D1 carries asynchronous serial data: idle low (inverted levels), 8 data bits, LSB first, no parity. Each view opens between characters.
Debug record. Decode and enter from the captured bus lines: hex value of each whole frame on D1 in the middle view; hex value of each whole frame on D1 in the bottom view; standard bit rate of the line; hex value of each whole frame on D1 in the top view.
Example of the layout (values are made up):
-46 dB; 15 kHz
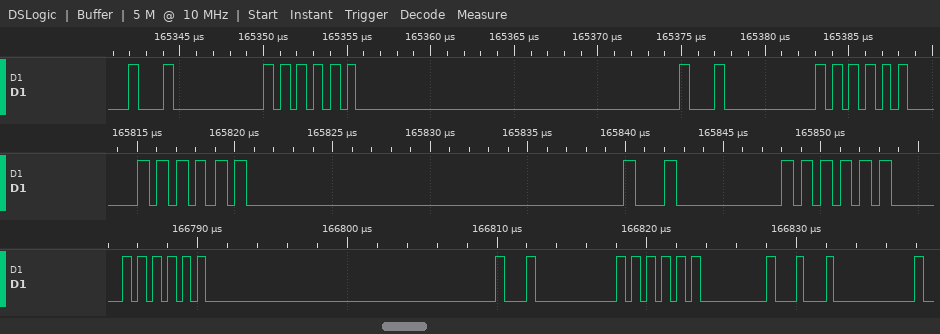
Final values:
55, FF, F7, 55; 55, FF, F7, 55, FF, 77; 2000000 baud; F7, 55, FF, F7, 55
